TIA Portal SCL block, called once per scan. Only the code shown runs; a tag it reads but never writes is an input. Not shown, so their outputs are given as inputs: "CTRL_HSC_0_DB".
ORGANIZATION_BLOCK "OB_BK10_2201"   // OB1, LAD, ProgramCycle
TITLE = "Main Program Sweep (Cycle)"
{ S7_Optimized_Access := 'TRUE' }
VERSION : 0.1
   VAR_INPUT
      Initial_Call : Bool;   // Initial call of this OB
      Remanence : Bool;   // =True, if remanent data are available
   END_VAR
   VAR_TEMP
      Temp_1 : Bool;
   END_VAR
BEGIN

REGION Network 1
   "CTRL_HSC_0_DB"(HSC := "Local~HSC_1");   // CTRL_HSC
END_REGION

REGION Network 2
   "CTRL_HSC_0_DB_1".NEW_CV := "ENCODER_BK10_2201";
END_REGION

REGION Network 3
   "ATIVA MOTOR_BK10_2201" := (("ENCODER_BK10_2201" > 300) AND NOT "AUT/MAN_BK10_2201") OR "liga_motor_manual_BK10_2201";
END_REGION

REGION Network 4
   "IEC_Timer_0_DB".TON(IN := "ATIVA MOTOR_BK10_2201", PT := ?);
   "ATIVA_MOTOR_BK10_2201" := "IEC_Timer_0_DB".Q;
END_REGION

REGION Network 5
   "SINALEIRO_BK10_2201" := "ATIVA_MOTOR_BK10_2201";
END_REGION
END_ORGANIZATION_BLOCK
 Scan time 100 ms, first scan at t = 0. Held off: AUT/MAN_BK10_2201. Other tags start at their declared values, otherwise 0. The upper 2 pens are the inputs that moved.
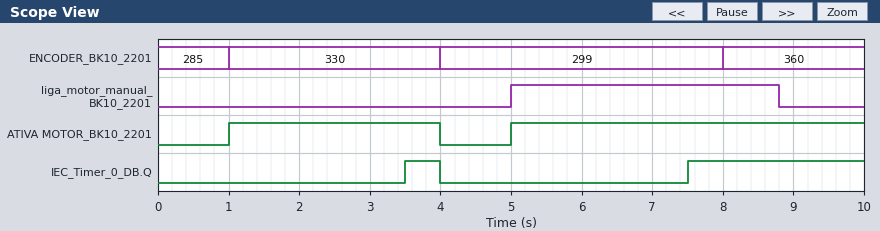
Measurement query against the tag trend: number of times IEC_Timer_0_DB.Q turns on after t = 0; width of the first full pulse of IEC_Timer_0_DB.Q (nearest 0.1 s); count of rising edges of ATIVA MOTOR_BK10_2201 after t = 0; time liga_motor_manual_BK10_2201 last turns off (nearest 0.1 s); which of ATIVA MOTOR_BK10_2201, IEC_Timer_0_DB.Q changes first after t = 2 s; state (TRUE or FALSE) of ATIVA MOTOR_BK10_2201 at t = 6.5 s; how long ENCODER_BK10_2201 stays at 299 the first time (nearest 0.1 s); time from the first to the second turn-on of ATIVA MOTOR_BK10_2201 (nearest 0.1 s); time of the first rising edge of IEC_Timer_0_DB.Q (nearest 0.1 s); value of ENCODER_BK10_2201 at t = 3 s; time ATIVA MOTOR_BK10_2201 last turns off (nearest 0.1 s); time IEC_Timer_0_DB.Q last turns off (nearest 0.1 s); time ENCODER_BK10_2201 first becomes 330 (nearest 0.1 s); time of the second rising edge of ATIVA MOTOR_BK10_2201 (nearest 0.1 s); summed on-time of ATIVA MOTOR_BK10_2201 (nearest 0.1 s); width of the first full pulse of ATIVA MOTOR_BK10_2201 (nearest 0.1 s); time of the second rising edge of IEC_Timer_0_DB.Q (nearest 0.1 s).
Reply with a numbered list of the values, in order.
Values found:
1. 2
2. 0.5 s
3. 2
4. 8.8 s
5. IEC_Timer_0_DB.Q
6. TRUE
7. 4.0 s
8. 4.0 s
9. 3.5 s
10. 330
11. 4.0 s
12. 4.0 s
13. 1.0 s
14. 5.0 s
15. 8.0 s
16. 3.0 s
17. 7.5 s
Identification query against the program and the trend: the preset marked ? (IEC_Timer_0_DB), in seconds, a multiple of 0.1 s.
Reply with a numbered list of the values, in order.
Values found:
1. 2.5 s
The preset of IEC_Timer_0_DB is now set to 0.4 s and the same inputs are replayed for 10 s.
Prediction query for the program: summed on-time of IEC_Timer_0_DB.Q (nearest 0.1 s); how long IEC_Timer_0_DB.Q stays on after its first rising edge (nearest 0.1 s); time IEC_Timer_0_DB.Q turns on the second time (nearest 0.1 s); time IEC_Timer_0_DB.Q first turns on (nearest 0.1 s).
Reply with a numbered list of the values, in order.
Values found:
1. 7.2 s
2. 2.6 s
3. 5.4 s
4. 1.4 s
